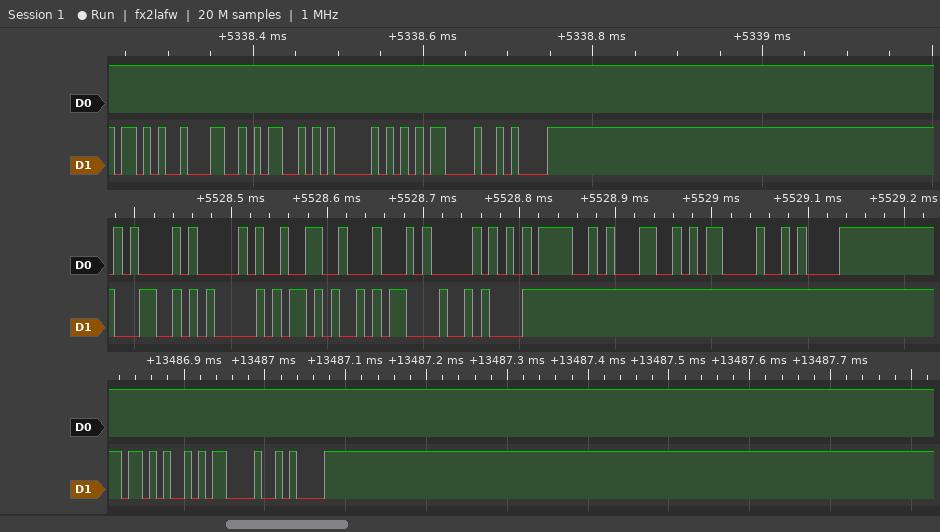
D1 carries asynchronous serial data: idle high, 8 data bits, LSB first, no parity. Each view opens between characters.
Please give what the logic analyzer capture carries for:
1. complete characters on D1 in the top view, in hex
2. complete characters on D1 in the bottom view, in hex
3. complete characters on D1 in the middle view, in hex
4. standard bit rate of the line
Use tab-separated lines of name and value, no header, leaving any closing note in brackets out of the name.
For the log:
complete characters on D1 in the top view, in hex	2B, 4C, 53, 50, 0D, 0A
complete characters on D1 in the bottom view, in hex	2B, 0D, 0A
complete characters on D1 in the middle view, in hex	4C, 41, 2B, 0D, 0A
standard bit rate of the line	115200 baud
